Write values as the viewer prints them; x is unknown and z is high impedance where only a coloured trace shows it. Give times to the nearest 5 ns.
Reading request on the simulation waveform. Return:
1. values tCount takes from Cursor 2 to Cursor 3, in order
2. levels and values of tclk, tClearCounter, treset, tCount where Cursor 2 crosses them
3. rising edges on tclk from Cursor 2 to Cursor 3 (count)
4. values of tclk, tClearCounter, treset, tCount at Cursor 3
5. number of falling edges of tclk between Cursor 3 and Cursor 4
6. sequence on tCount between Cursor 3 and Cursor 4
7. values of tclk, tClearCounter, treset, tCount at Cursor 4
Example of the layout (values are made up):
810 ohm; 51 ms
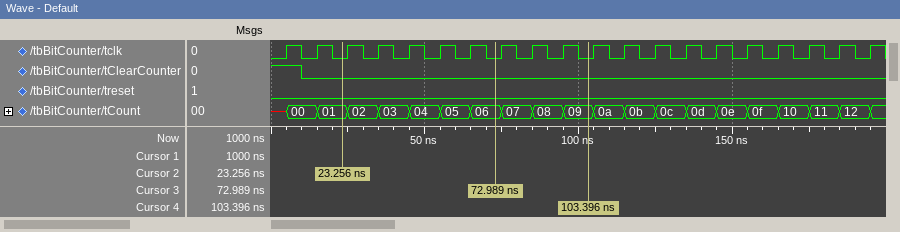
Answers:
01, 02, 03, 04, 05, 06; tclk=0, tClearCounter=0, treset=0, tCount=01; 5; tclk=0, tClearCounter=0, treset=0, tCount=06; 3; 06, 07, 08, 09; tclk=0, tClearCounter=0, treset=0, tCount=09
